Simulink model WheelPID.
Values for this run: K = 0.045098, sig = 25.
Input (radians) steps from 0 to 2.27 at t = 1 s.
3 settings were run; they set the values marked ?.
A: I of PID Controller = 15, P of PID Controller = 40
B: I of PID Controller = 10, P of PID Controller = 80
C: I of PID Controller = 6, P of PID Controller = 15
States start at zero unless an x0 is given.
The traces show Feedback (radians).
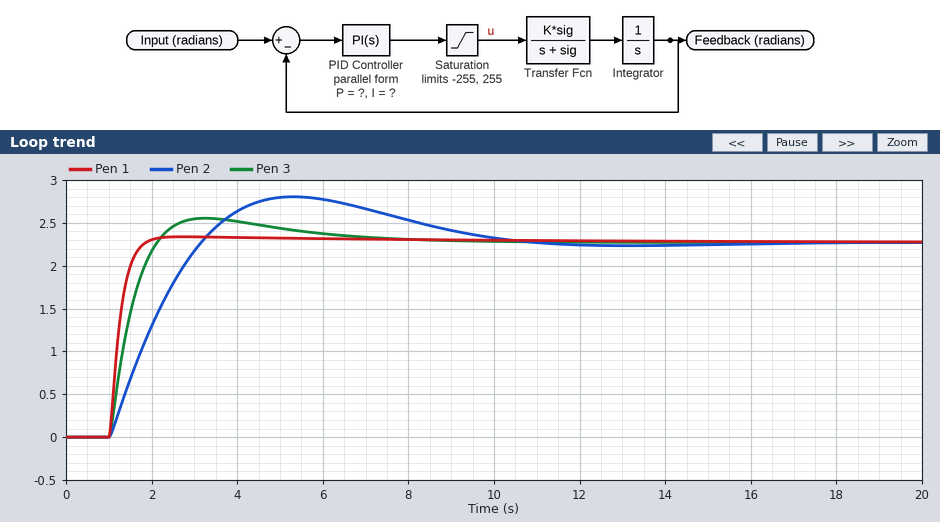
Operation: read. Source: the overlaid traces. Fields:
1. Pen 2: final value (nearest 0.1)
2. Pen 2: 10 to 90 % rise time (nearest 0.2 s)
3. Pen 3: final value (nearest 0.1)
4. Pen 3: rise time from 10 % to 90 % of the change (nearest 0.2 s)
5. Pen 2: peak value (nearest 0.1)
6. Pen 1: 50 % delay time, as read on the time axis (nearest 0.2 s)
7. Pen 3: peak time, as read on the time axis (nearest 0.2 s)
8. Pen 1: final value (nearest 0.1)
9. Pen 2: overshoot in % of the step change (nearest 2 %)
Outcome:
2.3
1.6 s
2.3
0.8 s
2.8
1.2 s
3.2 s
2.3
24 %
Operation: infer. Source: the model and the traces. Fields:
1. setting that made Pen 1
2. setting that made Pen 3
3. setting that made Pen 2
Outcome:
B
A
C
